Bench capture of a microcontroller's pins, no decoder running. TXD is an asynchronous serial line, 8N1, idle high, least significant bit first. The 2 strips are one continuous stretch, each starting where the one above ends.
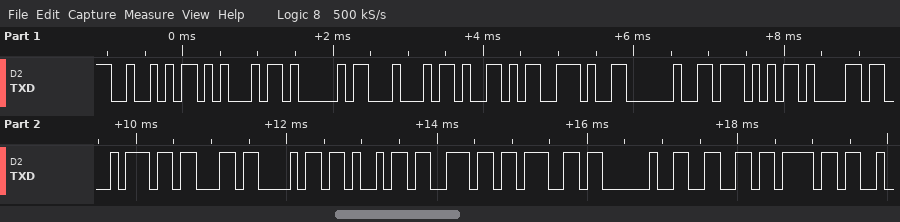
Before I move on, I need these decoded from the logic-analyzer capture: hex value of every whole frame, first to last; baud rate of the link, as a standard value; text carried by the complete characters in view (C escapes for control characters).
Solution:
52 45 41 44 59 2E 20 57 61 74 63 68 69 6E 67 20 66 6F
9600 baud
"READY. Watching fo"
